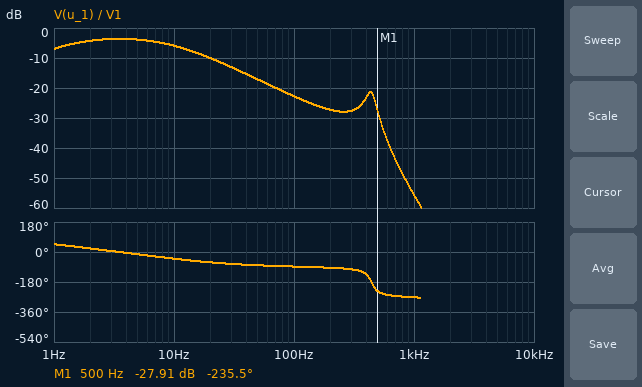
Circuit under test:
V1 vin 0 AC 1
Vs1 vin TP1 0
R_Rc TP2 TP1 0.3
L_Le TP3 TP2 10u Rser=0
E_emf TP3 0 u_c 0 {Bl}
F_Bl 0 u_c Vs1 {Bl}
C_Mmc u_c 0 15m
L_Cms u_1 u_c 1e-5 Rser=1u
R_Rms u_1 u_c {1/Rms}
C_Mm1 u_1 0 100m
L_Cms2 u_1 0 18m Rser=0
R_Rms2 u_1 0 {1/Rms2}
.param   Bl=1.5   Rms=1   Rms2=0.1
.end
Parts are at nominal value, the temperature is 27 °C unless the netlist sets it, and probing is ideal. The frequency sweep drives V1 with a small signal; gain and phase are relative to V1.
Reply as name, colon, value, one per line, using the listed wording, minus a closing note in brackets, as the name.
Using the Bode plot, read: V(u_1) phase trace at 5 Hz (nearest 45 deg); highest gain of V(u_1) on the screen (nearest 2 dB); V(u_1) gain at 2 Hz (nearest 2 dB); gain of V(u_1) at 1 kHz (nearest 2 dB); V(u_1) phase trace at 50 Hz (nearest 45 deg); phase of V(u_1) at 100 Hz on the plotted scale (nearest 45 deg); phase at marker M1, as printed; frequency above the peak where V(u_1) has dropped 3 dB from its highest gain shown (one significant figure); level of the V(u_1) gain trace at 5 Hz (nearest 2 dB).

V(u_1) phase trace at 5 Hz: 0 deg
highest gain of V(u_1) on the screen: -4 dB
V(u_1) gain at 2 Hz: -4 dB
gain of V(u_1) at 1 kHz: -56 dB
V(u_1) phase trace at 50 Hz: -90 deg
phase of V(u_1) at 100 Hz on the plotted scale: -90 deg
phase at marker M1, as printed: -235.5 deg
frequency above the peak where V(u_1) has dropped 3 dB from its highest gain shown: 10 Hz
level of the V(u_1) gain trace at 5 Hz: -4 dB
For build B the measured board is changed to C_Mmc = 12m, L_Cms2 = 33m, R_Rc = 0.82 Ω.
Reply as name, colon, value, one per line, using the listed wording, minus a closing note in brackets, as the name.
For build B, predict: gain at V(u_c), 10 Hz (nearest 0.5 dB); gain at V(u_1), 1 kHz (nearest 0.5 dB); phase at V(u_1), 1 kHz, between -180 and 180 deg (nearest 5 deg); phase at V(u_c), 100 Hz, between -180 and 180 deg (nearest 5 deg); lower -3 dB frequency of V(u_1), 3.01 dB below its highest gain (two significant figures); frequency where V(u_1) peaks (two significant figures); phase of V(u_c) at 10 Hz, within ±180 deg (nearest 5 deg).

gain at V(u_c), 10 Hz: -12.0 dB
gain at V(u_1), 1 kHz: -62.0 dB
phase at V(u_1), 1 kHz, between -180 and 180 deg: 95 deg
phase at V(u_c), 100 Hz, between -180 and 180 deg: -90 deg
lower -3 dB frequency of V(u_1), 3.01 dB below its highest gain: 1.3 Hz
frequency where V(u_1) peaks: 2.6 Hz
phase of V(u_c) at 10 Hz, within ±180 deg: -65 deg
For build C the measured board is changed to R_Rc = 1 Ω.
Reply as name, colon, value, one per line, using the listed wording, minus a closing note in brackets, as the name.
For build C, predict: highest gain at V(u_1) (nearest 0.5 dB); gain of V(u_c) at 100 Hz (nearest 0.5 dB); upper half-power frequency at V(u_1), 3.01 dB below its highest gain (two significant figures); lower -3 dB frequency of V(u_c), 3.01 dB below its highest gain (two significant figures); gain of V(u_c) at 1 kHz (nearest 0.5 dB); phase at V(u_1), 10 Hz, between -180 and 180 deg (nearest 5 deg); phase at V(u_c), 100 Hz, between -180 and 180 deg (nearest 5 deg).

highest gain at V(u_1): -4.0 dB
gain of V(u_c) at 100 Hz: -37.5 dB
upper half-power frequency at V(u_1), 3.01 dB below its highest gain: 5.5 Hz
lower -3 dB frequency of V(u_c), 3.01 dB below its highest gain: 2.2 Hz
gain of V(u_c) at 1 kHz: -34.5 dB
phase at V(u_1), 10 Hz, between -180 and 180 deg: -70 deg
phase at V(u_c), 100 Hz, between -180 and 180 deg: -90 deg
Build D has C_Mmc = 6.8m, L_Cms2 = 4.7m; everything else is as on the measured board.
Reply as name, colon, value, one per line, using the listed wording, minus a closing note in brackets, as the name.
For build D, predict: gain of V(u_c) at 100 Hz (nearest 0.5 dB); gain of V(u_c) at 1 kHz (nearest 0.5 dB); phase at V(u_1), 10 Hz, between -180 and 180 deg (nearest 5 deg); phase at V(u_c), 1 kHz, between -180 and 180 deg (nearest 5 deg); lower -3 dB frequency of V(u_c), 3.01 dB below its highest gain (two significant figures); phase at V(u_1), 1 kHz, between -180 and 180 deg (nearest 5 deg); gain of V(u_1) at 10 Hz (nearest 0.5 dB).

gain of V(u_c) at 100 Hz: -26.5 dB
gain of V(u_c) at 1 kHz: -14.5 dB
phase at V(u_1), 10 Hz, between -180 and 180 deg: -25 deg
phase at V(u_c), 1 kHz, between -180 and 180 deg: -85 deg
lower -3 dB frequency of V(u_c), 3.01 dB below its highest gain: 3.4 Hz
phase at V(u_1), 1 kHz, between -180 and 180 deg: 100 deg
gain of V(u_1) at 10 Hz: -4.5 dB
